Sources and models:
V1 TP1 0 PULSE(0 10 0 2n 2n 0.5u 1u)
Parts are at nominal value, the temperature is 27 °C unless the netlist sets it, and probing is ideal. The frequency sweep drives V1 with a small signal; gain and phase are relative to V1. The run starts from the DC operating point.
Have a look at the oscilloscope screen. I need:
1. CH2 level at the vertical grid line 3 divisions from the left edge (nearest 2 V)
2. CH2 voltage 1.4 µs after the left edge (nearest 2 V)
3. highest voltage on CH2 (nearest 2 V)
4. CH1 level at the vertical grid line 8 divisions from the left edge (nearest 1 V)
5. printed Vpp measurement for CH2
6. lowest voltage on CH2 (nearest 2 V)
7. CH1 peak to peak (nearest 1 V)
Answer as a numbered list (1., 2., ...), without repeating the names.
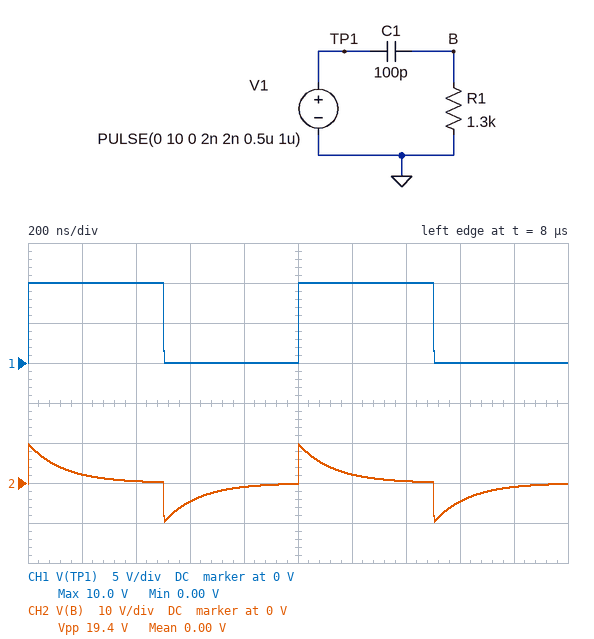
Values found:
1. -4 V
2. 0 V
3. 10 V
4. 0 V
5. 19.4 V
6. -10 V
7. 10 V
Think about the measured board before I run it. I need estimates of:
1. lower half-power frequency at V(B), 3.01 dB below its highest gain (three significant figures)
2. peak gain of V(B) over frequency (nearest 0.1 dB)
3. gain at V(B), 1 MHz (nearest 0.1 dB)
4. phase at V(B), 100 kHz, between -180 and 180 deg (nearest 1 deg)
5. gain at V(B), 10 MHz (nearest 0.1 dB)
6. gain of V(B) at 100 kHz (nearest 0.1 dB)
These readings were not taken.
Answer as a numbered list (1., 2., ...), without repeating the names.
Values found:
1. 1.22 MHz
2. 0 dB
3. -4.0 dB
4. 85 deg
5. -0.1 dB
6. -21.8 dB
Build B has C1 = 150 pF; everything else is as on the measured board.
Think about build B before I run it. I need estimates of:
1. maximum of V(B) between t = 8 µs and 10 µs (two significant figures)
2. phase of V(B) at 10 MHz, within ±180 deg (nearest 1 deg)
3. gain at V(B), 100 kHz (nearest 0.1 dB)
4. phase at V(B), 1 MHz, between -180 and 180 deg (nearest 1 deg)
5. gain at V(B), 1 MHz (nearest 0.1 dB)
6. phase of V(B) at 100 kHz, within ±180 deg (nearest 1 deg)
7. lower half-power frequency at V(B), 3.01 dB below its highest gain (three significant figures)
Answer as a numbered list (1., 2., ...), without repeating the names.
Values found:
1. 9.2 V
2. 5 deg
3. -18.3 dB
4. 39 deg
5. -2.2 dB
6. 83 deg
7. 816 kHz
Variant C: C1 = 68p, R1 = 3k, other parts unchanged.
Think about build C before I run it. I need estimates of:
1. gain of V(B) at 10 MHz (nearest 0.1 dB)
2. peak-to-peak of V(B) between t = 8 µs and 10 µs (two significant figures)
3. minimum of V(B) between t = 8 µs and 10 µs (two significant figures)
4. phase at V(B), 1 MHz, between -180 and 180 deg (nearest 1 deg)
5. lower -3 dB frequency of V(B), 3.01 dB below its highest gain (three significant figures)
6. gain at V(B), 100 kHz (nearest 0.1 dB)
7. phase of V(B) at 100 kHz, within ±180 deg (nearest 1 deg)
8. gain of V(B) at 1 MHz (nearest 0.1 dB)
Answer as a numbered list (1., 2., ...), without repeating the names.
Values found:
1. 0 dB
2. 18 V
3. -9.2 V
4. 38 deg
5. 780 kHz
6. -17.9 dB
7. 83 deg
8. -2.1 dB
